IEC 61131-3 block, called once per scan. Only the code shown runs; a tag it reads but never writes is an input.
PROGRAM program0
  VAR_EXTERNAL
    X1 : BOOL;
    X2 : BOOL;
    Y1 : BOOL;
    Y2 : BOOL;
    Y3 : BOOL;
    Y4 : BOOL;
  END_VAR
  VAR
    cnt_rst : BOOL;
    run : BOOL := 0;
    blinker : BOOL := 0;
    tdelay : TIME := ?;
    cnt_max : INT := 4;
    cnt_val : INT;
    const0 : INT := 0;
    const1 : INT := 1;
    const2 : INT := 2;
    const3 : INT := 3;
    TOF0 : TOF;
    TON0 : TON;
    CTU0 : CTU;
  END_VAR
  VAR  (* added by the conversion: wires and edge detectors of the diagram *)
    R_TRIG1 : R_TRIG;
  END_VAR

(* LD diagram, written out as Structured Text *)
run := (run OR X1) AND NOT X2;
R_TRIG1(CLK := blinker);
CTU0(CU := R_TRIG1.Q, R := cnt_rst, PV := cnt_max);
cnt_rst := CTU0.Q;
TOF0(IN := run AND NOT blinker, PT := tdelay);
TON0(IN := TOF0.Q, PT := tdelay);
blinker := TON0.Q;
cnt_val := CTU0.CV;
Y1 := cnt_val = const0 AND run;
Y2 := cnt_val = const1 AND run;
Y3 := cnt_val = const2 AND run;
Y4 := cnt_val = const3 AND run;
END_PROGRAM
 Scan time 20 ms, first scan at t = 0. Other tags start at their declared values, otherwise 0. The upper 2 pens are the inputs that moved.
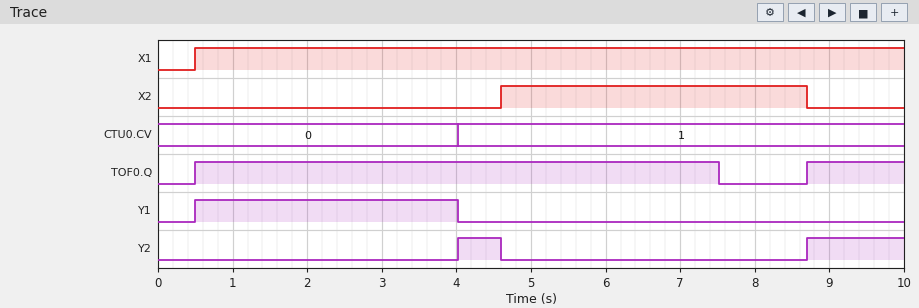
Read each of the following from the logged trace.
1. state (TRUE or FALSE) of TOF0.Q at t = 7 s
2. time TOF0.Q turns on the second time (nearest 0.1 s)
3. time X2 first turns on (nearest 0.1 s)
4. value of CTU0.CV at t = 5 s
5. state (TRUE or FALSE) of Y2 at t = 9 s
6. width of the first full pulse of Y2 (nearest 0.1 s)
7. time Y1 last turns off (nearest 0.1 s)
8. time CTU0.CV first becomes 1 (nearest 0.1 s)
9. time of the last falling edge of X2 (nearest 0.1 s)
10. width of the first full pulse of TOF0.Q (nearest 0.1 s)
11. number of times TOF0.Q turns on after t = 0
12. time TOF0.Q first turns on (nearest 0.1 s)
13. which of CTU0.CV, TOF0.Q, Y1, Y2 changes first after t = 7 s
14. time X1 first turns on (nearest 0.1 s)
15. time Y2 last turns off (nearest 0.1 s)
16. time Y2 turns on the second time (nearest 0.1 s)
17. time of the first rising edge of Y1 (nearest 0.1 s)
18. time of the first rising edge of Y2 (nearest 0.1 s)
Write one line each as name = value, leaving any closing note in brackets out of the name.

state (TRUE or FALSE) of TOF0.Q at t = 7 s = TRUE
time TOF0.Q turns on the second time = 8.7 s
time X2 first turns on = 4.6 s
value of CTU0.CV at t = 5 s = 1
state (TRUE or FALSE) of Y2 at t = 9 s = TRUE
width of the first full pulse of Y2 = 0.6 s
time Y1 last turns off = 4.0 s
time CTU0.CV first becomes 1 = 4.0 s
time of the last falling edge of X2 = 8.7 s
width of the first full pulse of TOF0.Q = 7.0 s
number of times TOF0.Q turns on after t = 0 = 2
time TOF0.Q first turns on = 0.5 s
which of CTU0.CV, TOF0.Q, Y1, Y2 changes first after t = 7 s = TOF0.Q
time X1 first turns on = 0.5 s
time Y2 last turns off = 4.6 s
time Y2 turns on the second time = 8.7 s
time of the first rising edge of Y1 = 0.5 s
time of the first rising edge of Y2 = 4.0 s
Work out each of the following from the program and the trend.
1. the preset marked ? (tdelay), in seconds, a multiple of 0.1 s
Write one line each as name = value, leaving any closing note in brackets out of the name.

the preset marked ? (tdelay), in seconds, a multiple of 0.1 s = 3.5 s
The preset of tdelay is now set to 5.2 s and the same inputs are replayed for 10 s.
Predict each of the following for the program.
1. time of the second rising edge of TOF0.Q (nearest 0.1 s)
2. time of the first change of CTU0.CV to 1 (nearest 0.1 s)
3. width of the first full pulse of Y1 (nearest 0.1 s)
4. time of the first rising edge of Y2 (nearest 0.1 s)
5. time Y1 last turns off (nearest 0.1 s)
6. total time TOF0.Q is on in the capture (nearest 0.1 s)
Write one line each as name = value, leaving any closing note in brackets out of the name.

time of the second rising edge of TOF0.Q = 9.8 s
time of the first change of CTU0.CV to 1 = 5.7 s
width of the first full pulse of Y1 = 4.1 s
time of the first rising edge of Y2 = 8.7 s
time Y1 last turns off = 4.6 s
total time TOF0.Q is on in the capture = 9.5 s
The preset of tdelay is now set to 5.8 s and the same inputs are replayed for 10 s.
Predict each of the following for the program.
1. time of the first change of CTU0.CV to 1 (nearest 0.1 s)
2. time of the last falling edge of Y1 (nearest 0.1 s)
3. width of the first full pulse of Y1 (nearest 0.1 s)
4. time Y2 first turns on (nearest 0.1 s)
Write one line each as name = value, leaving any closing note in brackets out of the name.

time of the first change of CTU0.CV to 1 = 6.3 s
time of the last falling edge of Y1 = 4.6 s
width of the first full pulse of Y1 = 4.1 s
time Y2 first turns on = 8.7 s
